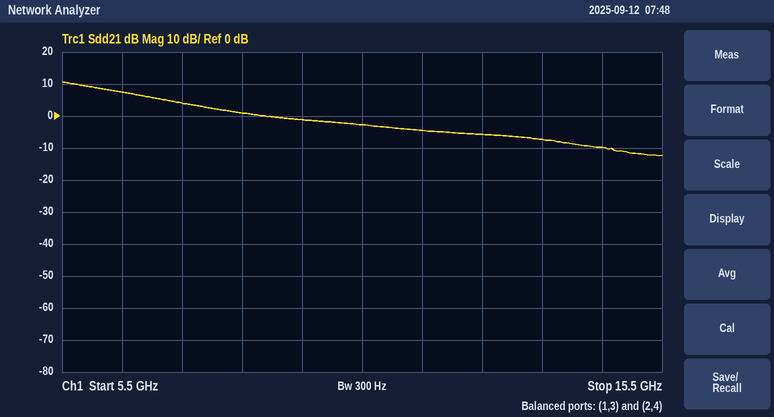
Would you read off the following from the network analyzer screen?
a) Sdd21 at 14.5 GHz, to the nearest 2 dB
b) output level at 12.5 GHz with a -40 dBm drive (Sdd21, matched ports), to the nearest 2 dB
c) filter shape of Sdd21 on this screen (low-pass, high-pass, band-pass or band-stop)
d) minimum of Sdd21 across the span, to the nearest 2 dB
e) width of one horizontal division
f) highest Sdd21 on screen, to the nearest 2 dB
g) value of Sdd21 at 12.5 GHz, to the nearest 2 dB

-10 dB
-46 dBm
low-pass
-12 dB
1 GHz
10 dB
-6 dB
